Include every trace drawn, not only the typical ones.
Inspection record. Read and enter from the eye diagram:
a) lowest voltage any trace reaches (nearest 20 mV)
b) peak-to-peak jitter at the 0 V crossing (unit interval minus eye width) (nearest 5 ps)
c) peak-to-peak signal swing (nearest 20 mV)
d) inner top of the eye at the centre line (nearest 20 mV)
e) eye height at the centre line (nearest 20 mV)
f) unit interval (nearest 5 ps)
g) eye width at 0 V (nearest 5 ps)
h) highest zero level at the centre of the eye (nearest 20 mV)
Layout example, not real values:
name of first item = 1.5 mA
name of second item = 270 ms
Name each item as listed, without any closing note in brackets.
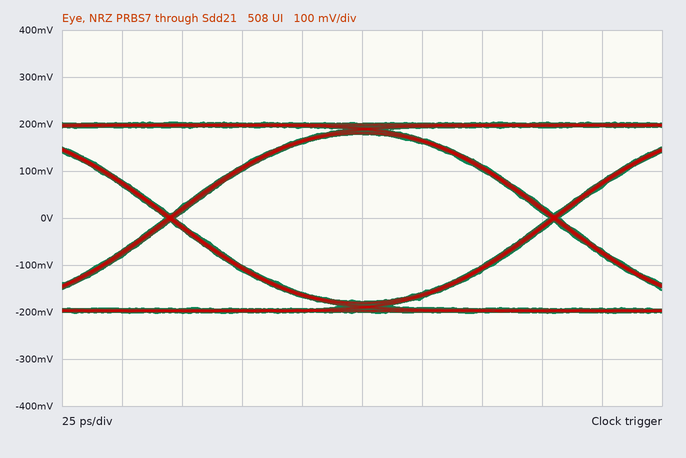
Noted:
lowest voltage any trace reaches = -200 mV
peak-to-peak jitter at the 0 V crossing (unit interval minus eye width) = 5 ps
peak-to-peak signal swing = 400 mV
inner top of the eye at the centre line = 180 mV
eye height at the centre line = 360 mV
unit interval = 160 ps
eye width at 0 V = 155 ps
highest zero level at the centre of the eye = -180 mV
